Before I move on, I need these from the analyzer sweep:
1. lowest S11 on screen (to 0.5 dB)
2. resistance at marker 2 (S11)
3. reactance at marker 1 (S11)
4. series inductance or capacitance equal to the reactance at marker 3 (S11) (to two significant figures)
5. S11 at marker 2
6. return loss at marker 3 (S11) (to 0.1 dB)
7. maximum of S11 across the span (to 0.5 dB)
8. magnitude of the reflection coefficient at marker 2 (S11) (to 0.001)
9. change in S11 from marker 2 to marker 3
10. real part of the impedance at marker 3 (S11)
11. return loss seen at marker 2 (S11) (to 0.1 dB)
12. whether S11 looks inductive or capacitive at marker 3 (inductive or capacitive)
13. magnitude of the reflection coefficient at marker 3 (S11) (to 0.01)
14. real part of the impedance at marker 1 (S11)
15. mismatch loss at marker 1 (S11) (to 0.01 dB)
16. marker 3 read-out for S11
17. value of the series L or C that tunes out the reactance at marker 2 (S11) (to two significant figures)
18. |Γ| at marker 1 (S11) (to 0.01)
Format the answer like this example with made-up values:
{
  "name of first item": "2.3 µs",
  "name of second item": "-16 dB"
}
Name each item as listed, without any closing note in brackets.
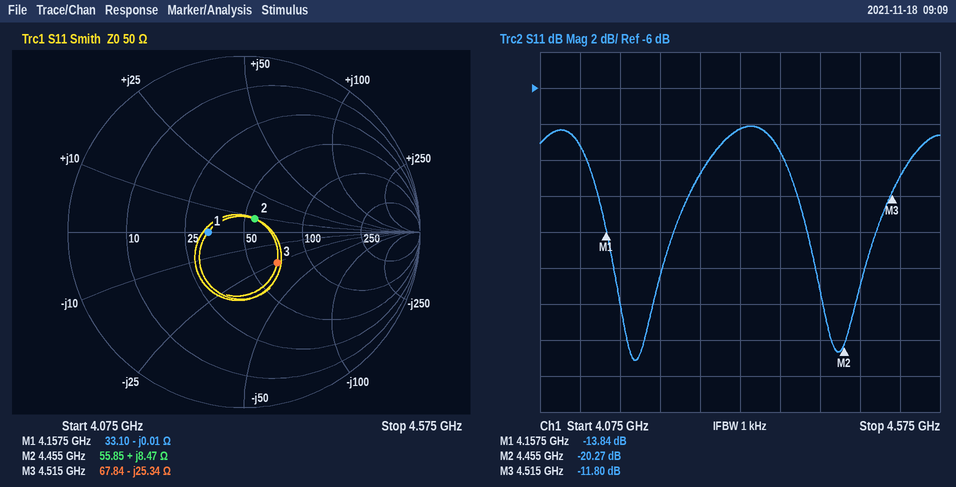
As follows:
{
  "lowest S11 on screen": "-21.0 dB",
  "resistance at marker 2": "55.85 Ω",
  "reactance at marker 1": "-0.01 Ω",
  "series inductance or capacitance equal to the reactance at marker 3 (S11)": "1.4 pF",
  "S11 at marker 2": "-20.27 dB",
  "return loss at marker 3 (S11)": "11.8 dB",
  "maximum of S11 across the span": "-8.0 dB",
  "magnitude of the reflection coefficient at marker 2 (S11)": "0.097",
  "change in S11 from marker 2 to marker 3": "8.47 dB",
  "real part of the impedance at marker 3": "67.84 Ω",
  "return loss seen at marker 2 (S11)": "20.3 dB",
  "whether S11 looks inductive or capacitive at marker 3": "capacitive",
  "magnitude of the reflection coefficient at marker 3 (S11)": "0.26",
  "real part of the impedance at marker 1": "33.10 Ω",
  "mismatch loss at marker 1 (S11)": "0.18 dB",
  "marker 3 read-out for S11": "-11.80 dB",
  "value of the series L or C that tunes out the reactance at marker 2 (S11)": "4.2 pF",
  "|Γ| at marker 1 (S11)": "0.20"
}
